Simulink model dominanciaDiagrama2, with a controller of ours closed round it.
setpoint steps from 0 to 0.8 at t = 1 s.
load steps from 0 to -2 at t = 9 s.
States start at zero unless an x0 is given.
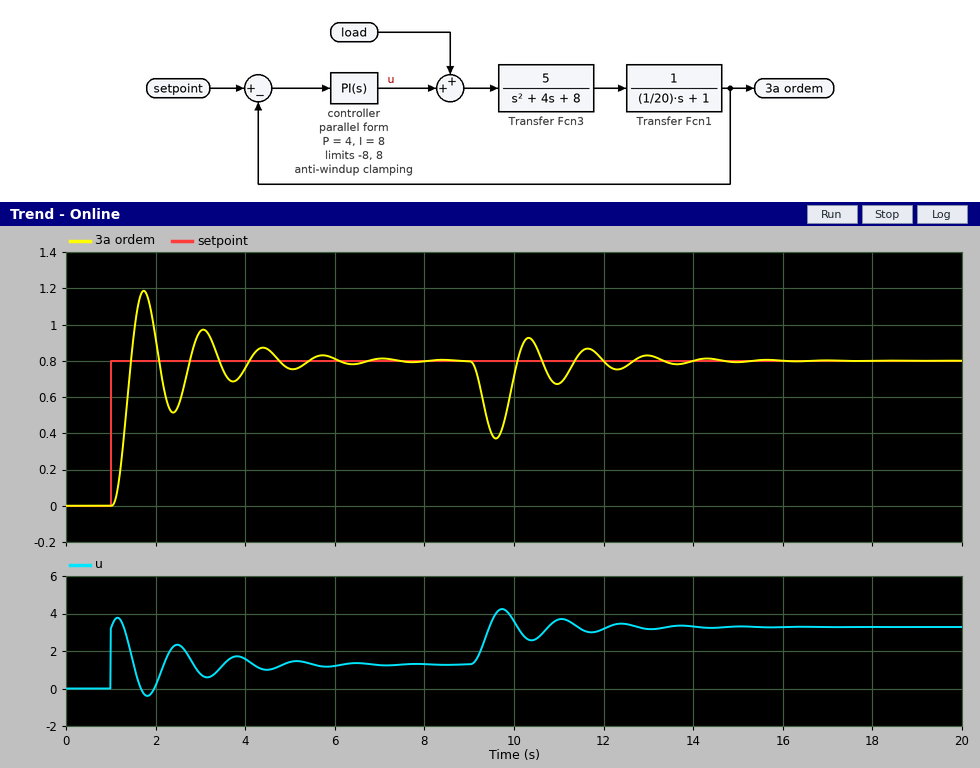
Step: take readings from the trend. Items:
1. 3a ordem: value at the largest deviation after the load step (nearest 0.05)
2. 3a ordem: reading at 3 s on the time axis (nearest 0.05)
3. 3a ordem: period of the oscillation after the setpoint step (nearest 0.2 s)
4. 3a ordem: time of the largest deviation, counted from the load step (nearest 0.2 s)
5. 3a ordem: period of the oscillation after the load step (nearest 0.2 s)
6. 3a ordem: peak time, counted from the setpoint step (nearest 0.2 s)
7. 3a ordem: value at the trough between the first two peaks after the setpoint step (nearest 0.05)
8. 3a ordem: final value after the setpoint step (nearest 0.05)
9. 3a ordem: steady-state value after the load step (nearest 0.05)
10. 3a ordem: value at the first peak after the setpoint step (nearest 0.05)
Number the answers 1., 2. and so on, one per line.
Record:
1. 0.35
2. 0.95
3. 1.4 s
4. 0.6 s
5. 1.4 s
6. 0.8 s
7. 0.50
8. 0.80
9. 0.80
10. 1.20
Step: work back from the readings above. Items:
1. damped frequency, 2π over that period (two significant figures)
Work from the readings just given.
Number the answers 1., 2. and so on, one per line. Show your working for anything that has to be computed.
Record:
1. 2π / 1.4 = 4.5 rad/s
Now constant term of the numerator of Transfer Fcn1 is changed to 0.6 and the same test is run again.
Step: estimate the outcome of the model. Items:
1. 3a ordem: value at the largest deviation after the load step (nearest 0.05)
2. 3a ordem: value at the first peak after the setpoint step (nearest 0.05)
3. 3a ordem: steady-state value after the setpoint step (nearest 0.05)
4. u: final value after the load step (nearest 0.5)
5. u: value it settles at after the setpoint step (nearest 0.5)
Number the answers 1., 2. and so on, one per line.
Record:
1. 0.45
2. 1.00
3. 0.80
4. 4.0
5. 2.0
